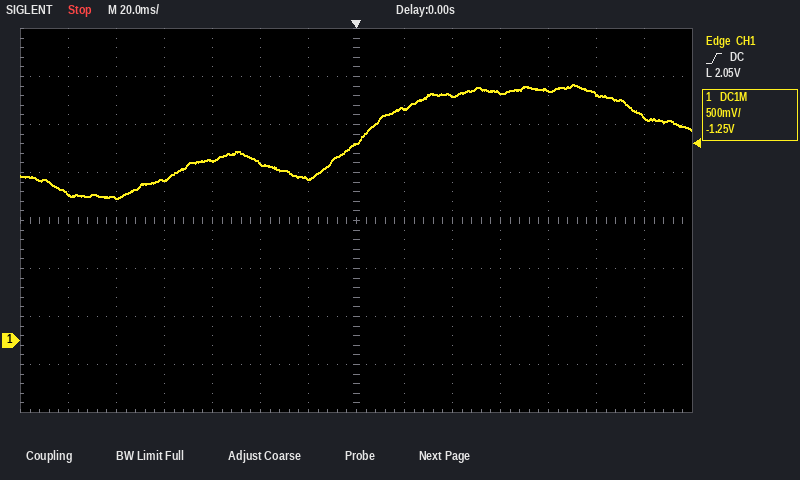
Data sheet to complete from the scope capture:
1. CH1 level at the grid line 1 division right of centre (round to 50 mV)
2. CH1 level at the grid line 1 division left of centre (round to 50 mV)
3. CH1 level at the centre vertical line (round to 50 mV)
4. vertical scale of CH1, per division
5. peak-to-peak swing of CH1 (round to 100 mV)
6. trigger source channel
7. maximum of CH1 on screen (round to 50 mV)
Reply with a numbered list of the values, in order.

1. 2.40 V
2. 1.70 V
3. 2.05 V
4. 500 mV
5. 1.20 V
6. CH1
7. 2.65 V
